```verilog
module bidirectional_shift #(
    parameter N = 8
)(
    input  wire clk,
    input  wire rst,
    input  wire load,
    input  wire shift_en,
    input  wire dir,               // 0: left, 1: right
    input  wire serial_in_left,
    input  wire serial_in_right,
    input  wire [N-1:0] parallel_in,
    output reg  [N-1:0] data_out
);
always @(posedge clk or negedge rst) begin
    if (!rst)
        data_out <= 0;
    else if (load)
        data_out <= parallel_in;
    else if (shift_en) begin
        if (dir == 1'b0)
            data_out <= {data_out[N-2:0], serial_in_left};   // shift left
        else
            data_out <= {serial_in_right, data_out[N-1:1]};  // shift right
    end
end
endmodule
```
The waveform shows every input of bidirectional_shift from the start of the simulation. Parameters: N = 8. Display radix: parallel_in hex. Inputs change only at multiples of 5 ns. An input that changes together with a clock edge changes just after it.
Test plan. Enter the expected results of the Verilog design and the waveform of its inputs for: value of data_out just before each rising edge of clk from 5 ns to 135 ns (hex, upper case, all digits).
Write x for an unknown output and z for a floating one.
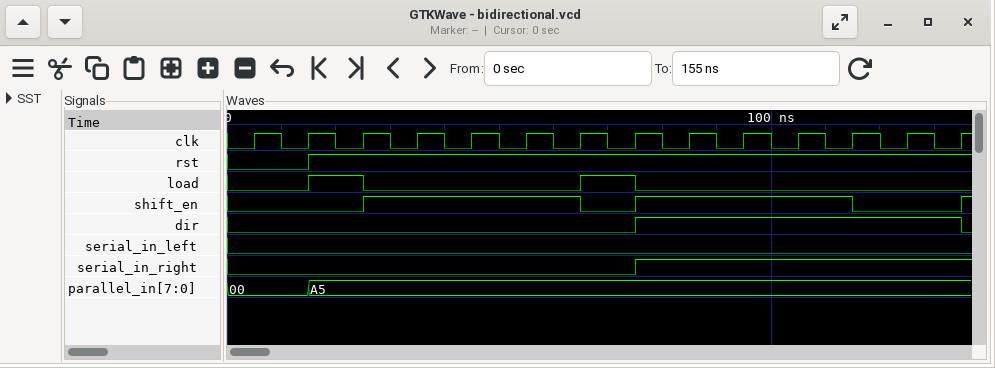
00, 00, 00, A5, 4A, 94, 28, 50, A5, D2, E9, F4, FA, FA
